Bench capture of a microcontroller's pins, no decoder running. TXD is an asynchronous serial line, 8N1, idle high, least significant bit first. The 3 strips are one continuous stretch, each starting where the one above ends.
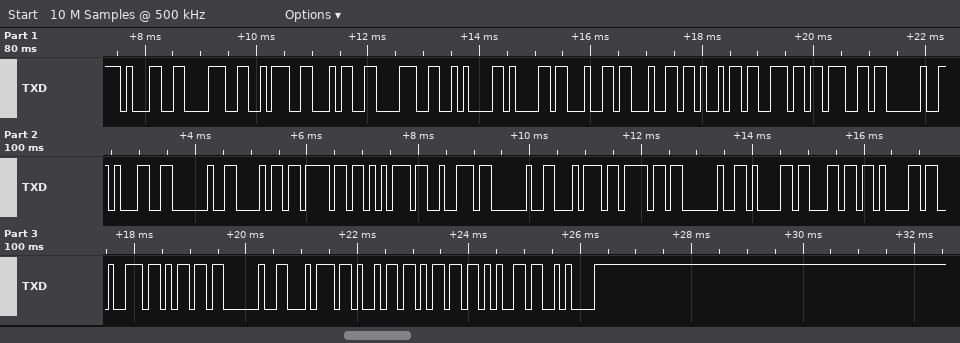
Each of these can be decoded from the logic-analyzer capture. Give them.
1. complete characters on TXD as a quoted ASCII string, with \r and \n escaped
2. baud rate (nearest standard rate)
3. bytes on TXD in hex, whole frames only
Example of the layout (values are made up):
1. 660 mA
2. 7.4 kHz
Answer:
1. "18:48\nadding 1 hour to alarm time\n"
2. 9600 baud
3. 31 38 3A 34 38 0A 61 64 64 69 6E 67 20 31 20 68 6F 75 72 20 74 6F 20 61 6C 61 72 6D 20 74 69 6D 65 0A
